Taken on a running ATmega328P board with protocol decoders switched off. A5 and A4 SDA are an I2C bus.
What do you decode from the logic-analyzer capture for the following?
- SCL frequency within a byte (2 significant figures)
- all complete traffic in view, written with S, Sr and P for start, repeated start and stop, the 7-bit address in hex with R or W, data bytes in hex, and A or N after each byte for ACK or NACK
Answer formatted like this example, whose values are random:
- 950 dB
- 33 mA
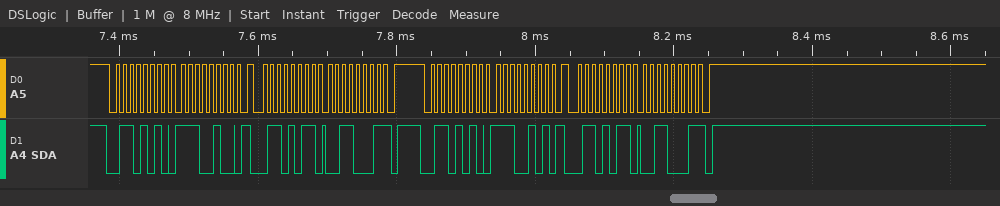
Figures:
- 100 kHz
- S 35W A E4 A Sr 35R A 31 N P S 35W A E5 A Sr 35R A 31 N P
